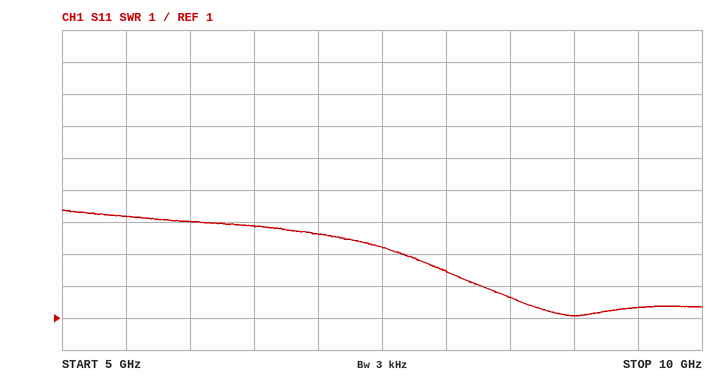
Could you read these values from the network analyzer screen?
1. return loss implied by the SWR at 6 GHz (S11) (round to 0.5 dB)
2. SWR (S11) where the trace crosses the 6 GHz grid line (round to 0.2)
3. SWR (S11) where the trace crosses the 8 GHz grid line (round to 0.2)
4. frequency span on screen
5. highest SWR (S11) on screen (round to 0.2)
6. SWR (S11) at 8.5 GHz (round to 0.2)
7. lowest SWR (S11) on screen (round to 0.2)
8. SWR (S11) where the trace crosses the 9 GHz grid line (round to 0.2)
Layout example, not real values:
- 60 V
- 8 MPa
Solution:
- 4.5 dB
- 4.0
- 2.4
- 5 GHz
- 4.4
- 1.6
- 1.0
- 1.0
